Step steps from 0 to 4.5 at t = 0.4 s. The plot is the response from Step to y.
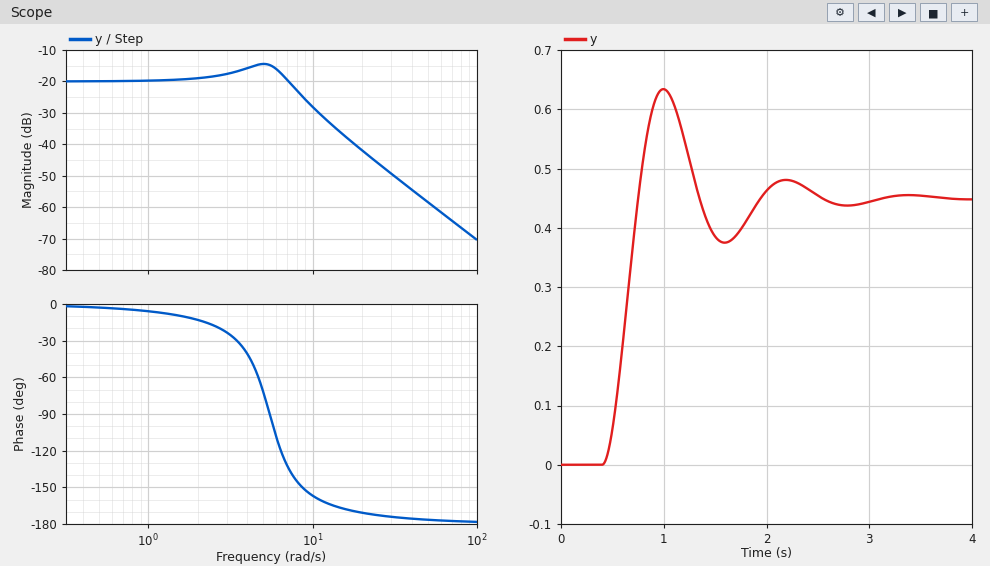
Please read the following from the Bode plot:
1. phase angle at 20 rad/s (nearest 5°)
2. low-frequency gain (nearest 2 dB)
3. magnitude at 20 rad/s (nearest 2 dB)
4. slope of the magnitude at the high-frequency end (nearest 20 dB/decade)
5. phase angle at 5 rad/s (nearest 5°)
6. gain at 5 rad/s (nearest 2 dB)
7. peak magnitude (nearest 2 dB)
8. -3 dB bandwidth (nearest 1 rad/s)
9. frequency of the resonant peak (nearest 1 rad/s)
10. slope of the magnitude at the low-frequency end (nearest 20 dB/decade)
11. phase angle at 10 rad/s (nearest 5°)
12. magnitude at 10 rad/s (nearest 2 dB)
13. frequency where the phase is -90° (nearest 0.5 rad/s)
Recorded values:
-170°
-20 dB
-42 dB
-40 dB/decade
-70°
-14 dB
-14 dB
8 rad/s
5 rad/s
0 dB/decade
-155°
-28 dB
5.5 rad/s
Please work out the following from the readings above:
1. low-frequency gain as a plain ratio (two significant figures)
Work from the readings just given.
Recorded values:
0.10
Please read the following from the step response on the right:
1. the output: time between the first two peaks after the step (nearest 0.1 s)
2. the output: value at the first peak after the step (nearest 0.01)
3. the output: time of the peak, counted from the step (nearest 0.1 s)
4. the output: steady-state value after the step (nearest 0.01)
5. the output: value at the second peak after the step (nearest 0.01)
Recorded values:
1.2 s
0.63
0.6 s
0.45
0.48
